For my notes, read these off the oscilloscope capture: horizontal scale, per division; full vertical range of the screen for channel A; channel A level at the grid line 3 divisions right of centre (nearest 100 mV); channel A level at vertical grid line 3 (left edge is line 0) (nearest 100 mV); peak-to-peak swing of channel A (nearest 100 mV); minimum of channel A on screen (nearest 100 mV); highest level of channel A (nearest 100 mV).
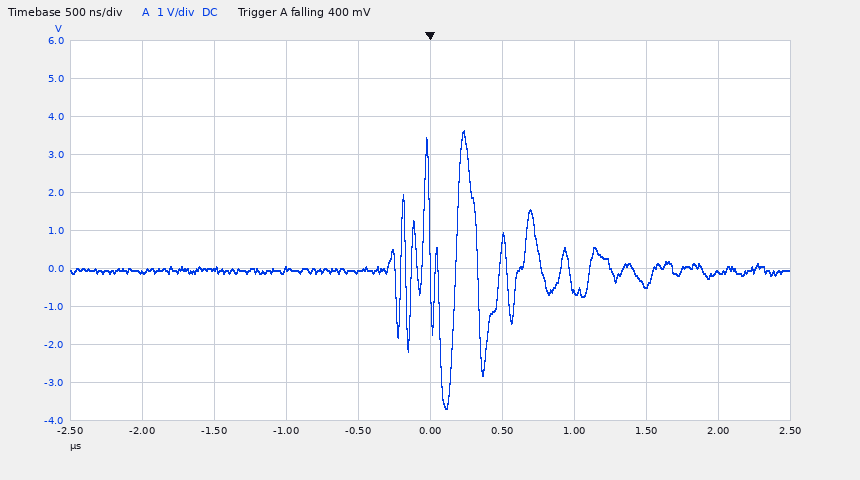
500 ns
10 V
-400 mV
0.0 V
7.3 V
-3.7 V
3.6 V
